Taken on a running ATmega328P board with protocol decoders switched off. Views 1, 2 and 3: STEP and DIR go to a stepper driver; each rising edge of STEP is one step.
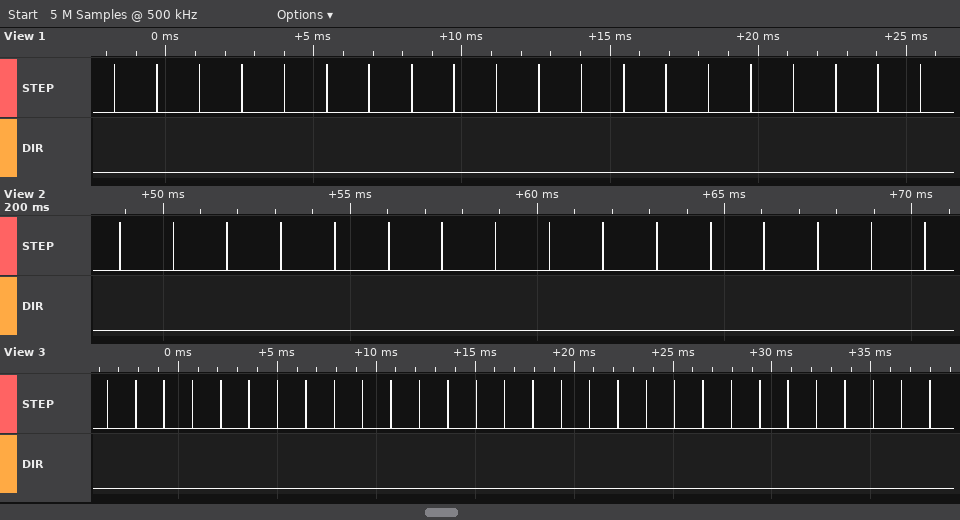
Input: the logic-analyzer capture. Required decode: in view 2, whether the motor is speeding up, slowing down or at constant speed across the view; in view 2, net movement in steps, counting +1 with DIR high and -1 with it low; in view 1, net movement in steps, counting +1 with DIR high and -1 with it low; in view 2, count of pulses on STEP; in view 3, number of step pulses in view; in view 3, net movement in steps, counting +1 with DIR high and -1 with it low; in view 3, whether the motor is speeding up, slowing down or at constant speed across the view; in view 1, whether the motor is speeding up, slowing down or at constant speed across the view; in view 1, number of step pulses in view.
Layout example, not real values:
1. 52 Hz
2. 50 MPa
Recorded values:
1. constant speed
2. -16
3. -20
4. 16
5. 30
6. -30
7. constant speed
8. constant speed
9. 20
